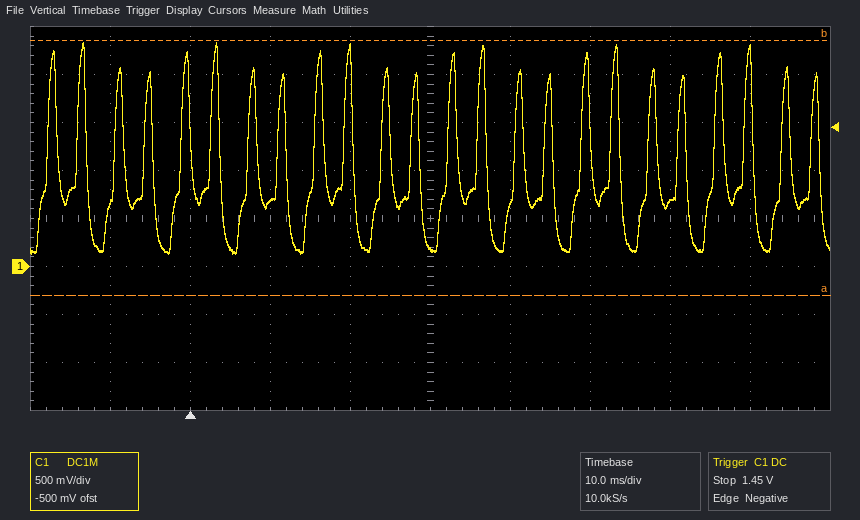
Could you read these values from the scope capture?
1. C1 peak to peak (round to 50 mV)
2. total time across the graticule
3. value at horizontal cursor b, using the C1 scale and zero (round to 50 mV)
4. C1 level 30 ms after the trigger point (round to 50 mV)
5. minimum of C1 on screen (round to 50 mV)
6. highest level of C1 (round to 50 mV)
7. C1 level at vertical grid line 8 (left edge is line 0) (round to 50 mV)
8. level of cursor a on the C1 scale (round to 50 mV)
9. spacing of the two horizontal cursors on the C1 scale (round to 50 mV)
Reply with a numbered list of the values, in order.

1. 2.20 V
2. 100 ms
3. 2.35 V
4. 200 mV
5. 150 mV
6. 2.35 V
7. 650 mV
8. -300 mV
9. 2.65 V
